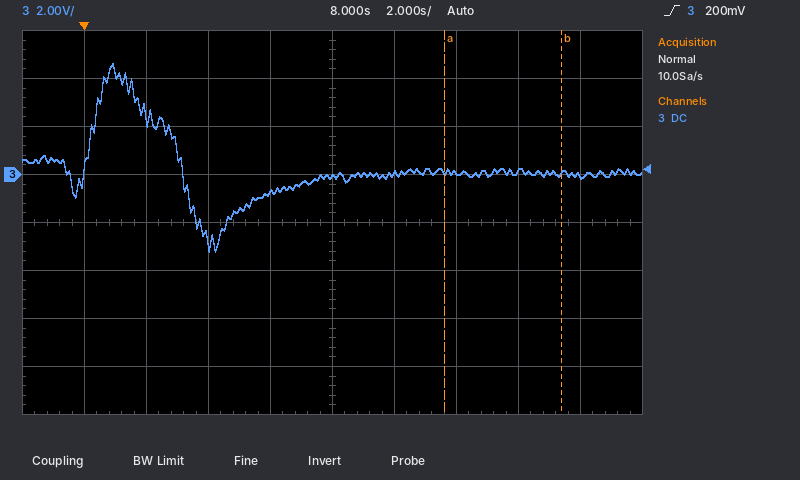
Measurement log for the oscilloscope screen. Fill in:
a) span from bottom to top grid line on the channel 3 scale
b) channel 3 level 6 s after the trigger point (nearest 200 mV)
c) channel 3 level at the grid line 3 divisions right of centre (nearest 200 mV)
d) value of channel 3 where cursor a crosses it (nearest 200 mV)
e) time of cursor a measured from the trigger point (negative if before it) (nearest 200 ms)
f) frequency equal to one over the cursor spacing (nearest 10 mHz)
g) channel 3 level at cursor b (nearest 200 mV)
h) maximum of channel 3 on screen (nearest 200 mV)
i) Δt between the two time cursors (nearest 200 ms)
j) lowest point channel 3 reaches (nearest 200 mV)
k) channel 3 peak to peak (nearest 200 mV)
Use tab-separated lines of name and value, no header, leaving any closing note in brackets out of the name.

span from bottom to top grid line on the channel 3 scale	16 V
channel 3 level 6 s after the trigger point	-800 mV
channel 3 level at the grid line 3 divisions right of centre	200 mV
value of channel 3 where cursor a crosses it	200 mV
time of cursor a measured from the trigger point (negative if before it)	+11.6 s
frequency equal to one over the cursor spacing	260 mHz
channel 3 level at cursor b	0.0 V
maximum of channel 3 on screen	4.6 V
Δt between the two time cursors	3.8 s
lowest point channel 3 reaches	-3.2 V
channel 3 peak to peak	7.8 V
